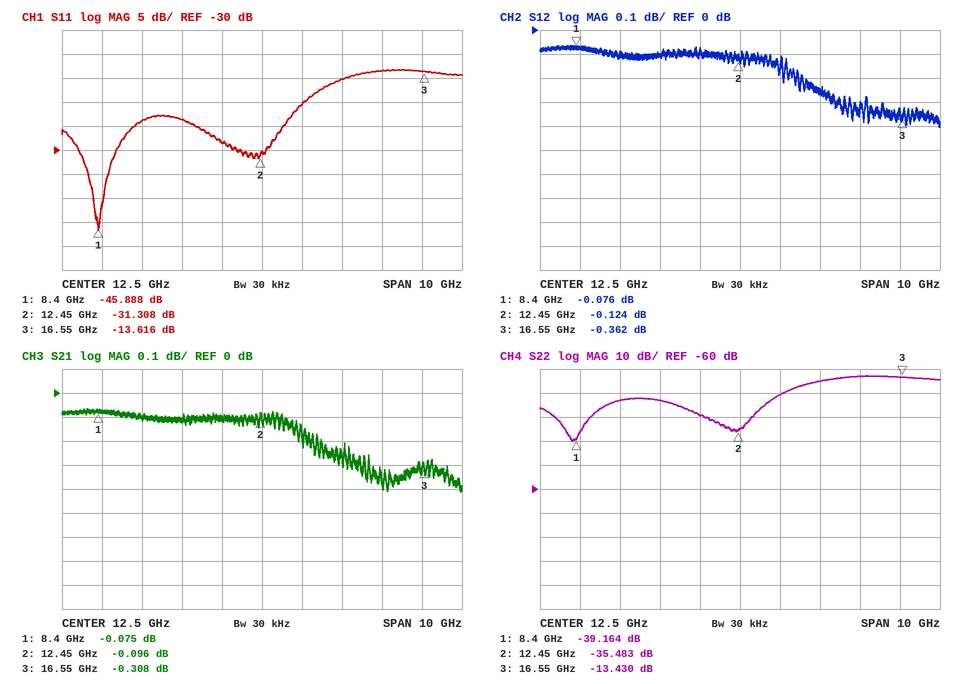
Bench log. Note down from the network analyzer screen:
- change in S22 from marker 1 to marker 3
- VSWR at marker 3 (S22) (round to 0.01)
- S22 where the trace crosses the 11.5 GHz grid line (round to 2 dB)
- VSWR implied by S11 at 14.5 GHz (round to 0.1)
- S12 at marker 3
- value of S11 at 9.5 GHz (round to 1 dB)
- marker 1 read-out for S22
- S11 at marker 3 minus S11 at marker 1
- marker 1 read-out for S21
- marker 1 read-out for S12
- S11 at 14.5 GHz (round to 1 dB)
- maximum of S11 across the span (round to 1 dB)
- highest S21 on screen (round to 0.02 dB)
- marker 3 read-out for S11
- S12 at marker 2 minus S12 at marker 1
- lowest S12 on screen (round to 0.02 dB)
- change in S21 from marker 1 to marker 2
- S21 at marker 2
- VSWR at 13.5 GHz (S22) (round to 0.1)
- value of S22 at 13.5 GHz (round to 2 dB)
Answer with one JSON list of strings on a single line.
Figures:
["25.734 dB", "1.54", "-30 dB", "1.4", "-0.362 dB", "-24 dB", "-39.164 dB", "32.272 dB", "-0.075 dB", "-0.076 dB", "-15 dB", "-13 dB", "-0.06 dB", "-13.616 dB", "-0.048 dB", "-0.40 dB", "-0.021 dB", "-0.096 dB", "1.2", "-20 dB"]
